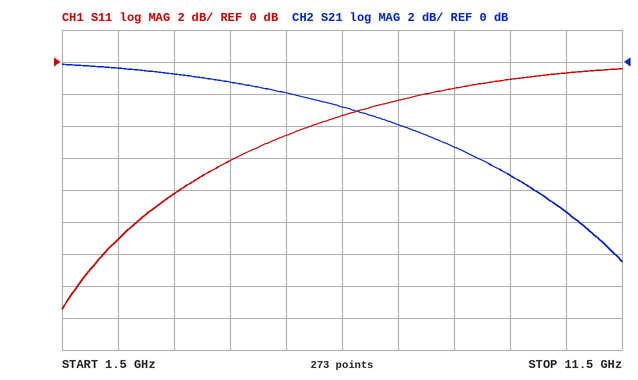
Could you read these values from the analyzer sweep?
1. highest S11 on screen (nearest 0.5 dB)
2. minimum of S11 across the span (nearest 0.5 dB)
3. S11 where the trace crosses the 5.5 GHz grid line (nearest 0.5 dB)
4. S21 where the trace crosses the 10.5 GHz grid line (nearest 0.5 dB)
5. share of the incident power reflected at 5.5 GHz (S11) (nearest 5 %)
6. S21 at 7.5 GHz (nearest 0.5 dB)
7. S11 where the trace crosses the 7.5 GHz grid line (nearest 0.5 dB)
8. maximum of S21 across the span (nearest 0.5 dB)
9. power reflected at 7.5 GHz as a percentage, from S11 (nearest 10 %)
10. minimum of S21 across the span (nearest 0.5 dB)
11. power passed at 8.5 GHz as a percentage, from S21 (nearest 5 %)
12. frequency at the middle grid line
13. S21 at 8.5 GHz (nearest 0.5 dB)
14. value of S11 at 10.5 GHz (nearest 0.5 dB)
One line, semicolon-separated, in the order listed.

-0.5 dB; -15.5 dB; -4.5 dB; -9.5 dB; 35 %; -4.0 dB; -2.5 dB; 0.0 dB; 60 %; -12.5 dB; 30 %; 6.5 GHz; -5.5 dB; -0.5 dB
